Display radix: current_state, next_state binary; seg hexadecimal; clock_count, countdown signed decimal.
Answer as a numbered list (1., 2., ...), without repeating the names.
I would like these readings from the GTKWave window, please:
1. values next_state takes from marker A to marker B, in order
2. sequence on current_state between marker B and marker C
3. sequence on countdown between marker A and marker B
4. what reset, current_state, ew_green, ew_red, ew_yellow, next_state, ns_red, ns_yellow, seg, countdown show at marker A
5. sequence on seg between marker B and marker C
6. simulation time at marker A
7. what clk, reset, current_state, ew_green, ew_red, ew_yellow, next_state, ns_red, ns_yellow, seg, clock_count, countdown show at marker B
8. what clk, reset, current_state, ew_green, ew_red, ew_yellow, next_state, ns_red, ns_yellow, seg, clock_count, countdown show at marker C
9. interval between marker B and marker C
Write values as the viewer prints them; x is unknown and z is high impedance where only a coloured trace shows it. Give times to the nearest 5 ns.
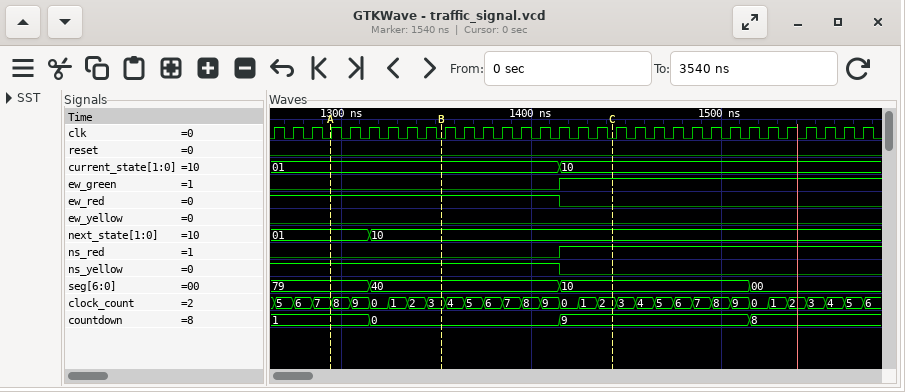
1. 01, 10
2. 01, 10
3. 1, 0
4. reset=0, current_state=01, ew_green=0, ew_red=1, ew_yellow=0, next_state=01, ns_red=0, ns_yellow=1, seg=79, countdown=1
5. 40, 10
6. 1295 ns
7. clk=0, reset=0, current_state=01, ew_green=0, ew_red=1, ew_yellow=0, next_state=10, ns_red=0, ns_yellow=1, seg=40, clock_count=3, countdown=0
8. clk=0, reset=0, current_state=10, ew_green=1, ew_red=0, ew_yellow=0, next_state=10, ns_red=1, ns_yellow=0, seg=10, clock_count=2, countdown=9
9. 90 ns
